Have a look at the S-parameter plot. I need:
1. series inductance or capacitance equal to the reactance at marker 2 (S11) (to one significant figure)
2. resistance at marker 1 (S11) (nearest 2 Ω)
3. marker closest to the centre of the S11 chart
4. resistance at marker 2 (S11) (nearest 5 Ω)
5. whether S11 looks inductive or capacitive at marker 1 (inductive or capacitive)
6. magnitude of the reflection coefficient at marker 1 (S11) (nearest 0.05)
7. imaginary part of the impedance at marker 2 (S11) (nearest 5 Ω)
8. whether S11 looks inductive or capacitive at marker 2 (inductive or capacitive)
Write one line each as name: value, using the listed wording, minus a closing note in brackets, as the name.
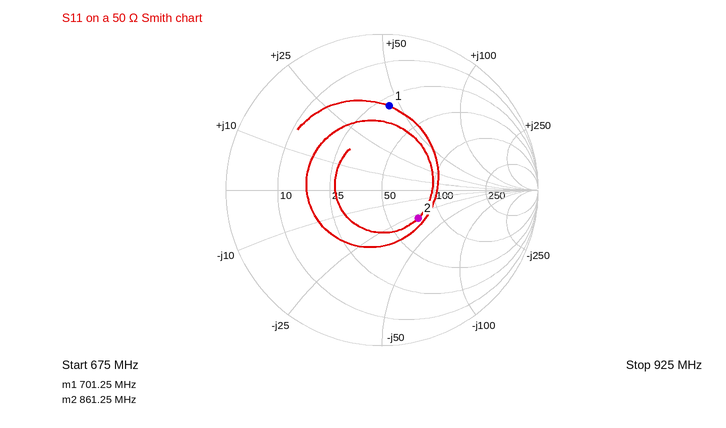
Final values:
series inductance or capacitance equal to the reactance at marker 2 (S11): 6 pF
resistance at marker 1 (S11): 30 Ω
marker closest to the centre of the S11 chart: marker 2
resistance at marker 2 (S11): 75 Ω
whether S11 looks inductive or capacitive at marker 1: inductive
magnitude of the reflection coefficient at marker 1 (S11): 0.55
imaginary part of the impedance at marker 2 (S11): -30 Ω
whether S11 looks inductive or capacitive at marker 2: capacitive
